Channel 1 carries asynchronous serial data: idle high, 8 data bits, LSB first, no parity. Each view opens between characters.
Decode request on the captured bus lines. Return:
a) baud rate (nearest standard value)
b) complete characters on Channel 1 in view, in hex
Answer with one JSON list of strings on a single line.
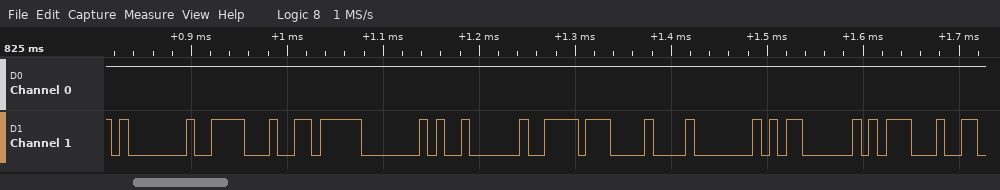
["115200 baud", "01, 1E, F6, 40, 02, DE, 08, 40, 03, 1D"]
